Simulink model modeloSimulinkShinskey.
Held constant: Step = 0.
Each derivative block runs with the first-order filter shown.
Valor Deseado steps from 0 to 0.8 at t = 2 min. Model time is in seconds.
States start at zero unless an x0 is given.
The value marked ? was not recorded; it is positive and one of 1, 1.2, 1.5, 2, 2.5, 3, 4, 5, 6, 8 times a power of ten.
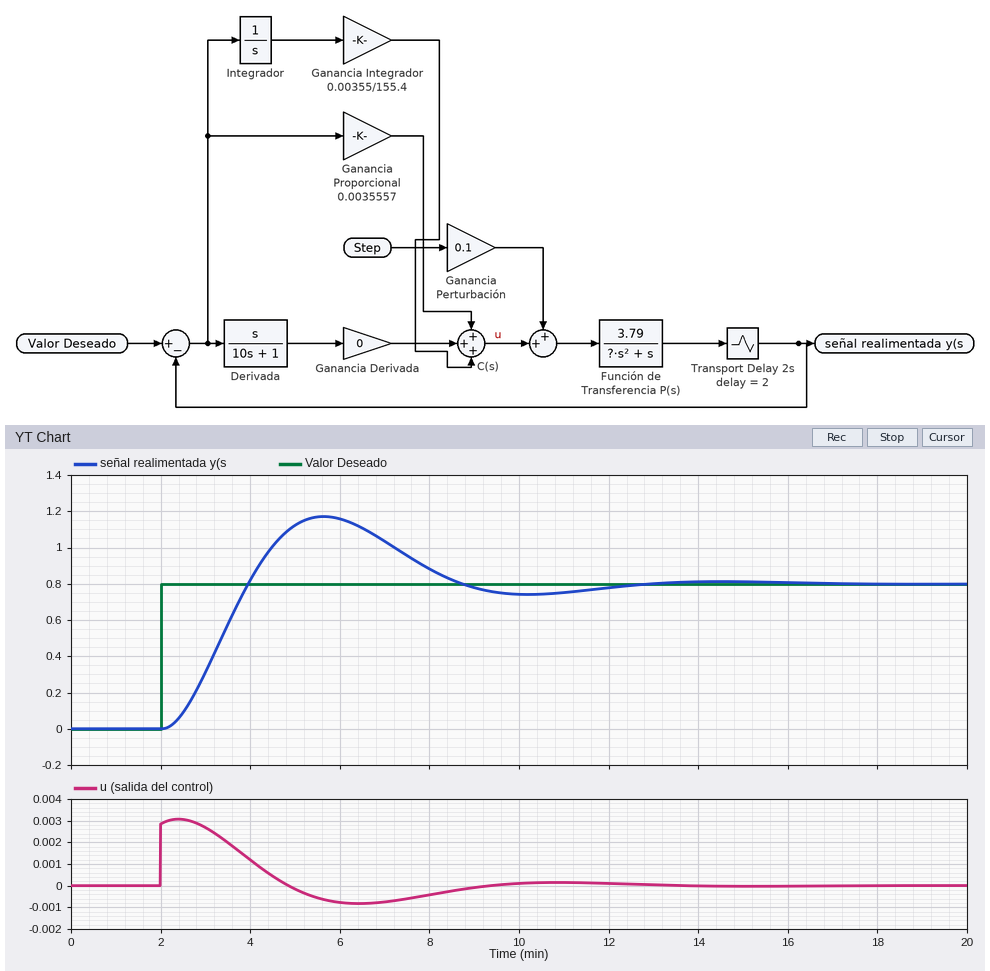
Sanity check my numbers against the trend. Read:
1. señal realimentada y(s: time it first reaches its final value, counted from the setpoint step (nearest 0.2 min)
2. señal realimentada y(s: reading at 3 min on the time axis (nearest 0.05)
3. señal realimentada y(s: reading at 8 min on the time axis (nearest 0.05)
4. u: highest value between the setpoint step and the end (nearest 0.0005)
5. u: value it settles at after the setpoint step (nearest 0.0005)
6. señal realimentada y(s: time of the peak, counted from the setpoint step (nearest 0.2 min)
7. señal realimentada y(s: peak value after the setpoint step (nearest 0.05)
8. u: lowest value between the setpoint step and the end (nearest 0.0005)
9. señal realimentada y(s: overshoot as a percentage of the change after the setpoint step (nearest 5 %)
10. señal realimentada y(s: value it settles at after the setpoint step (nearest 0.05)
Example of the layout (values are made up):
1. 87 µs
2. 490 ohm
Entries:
1. 2.0 min
2. 0.30
3. 0.90
4. 0.0030
5. 0.0000
6. 3.6 min
7. 1.15
8. -0.0010
9. 45 %
10. 0.80
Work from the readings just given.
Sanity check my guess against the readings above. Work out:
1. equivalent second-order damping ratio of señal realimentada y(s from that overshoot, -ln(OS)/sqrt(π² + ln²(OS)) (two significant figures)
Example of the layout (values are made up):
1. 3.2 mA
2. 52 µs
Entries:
1. 0.25
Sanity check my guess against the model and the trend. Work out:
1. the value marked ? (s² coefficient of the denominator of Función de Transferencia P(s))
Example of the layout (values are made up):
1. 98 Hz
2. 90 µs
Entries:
1. 40
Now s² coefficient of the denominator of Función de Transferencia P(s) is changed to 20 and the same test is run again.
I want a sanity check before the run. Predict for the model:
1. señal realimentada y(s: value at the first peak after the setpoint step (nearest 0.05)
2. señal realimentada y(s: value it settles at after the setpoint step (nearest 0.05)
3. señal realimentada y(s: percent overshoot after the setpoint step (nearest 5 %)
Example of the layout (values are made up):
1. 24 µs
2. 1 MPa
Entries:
1. 1.05
2. 0.80
3. 30 %
